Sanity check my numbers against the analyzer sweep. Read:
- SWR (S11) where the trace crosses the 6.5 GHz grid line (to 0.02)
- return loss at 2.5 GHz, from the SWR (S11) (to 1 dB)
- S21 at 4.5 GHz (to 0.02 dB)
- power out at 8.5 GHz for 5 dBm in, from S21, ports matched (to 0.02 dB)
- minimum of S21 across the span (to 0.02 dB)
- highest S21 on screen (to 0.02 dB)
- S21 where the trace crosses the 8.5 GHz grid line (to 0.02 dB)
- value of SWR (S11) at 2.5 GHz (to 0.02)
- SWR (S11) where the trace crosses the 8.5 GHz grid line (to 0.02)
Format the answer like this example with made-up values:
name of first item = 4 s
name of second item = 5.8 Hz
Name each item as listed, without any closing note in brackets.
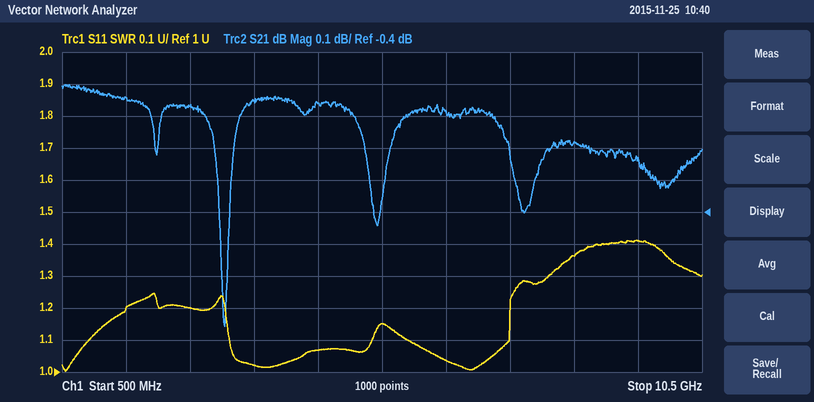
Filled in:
SWR (S11) where the trace crosses the 6.5 GHz grid line = 1.04
return loss at 2.5 GHz, from the SWR (S11) = 21 dB
S21 at 4.5 GHz = -0.06 dB
power out at 8.5 GHz for 5 dBm in, from S21, ports matched = 4.82 dBm
minimum of S21 across the span = -0.76 dB
highest S21 on screen = 0.00 dB
S21 where the trace crosses the 8.5 GHz grid line = -0.18 dB
value of SWR (S11) at 2.5 GHz = 1.20
SWR (S11) where the trace crosses the 8.5 GHz grid line = 1.36
